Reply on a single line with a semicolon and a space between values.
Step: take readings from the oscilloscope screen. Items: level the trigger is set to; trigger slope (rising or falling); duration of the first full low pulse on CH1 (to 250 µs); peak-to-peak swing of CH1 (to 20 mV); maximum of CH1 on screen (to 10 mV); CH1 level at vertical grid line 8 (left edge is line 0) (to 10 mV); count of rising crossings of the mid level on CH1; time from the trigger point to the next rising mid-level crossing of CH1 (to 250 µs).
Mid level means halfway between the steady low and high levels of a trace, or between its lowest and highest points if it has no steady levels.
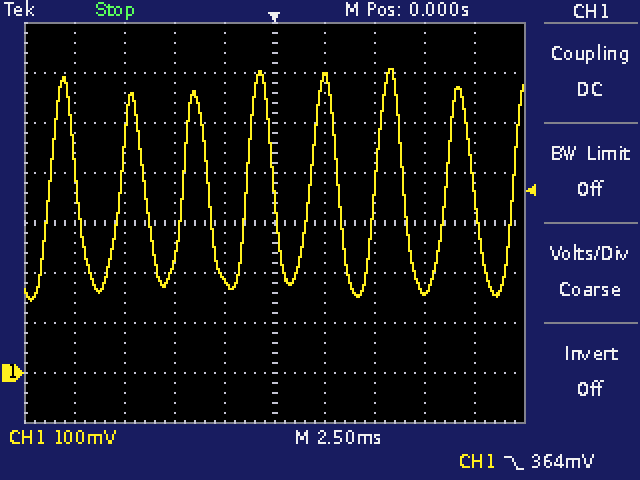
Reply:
364 mV; falling; 2.25 ms; 460 mV; 610 mV; 160 mV; 8; 1.75 ms
